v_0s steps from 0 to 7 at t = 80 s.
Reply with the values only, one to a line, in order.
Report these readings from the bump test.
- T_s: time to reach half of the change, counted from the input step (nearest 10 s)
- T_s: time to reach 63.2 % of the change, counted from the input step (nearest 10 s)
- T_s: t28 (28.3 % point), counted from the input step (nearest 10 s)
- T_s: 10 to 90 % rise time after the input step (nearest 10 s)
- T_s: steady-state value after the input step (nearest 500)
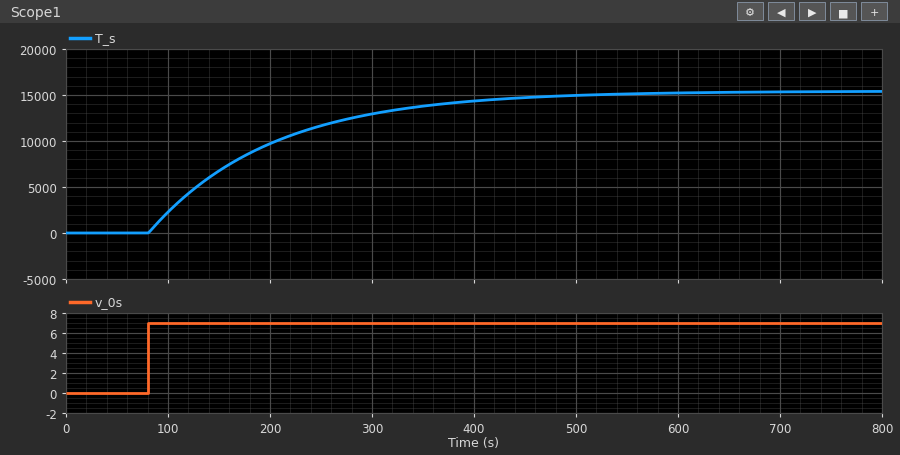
80 s
120 s
40 s
260 s
15500
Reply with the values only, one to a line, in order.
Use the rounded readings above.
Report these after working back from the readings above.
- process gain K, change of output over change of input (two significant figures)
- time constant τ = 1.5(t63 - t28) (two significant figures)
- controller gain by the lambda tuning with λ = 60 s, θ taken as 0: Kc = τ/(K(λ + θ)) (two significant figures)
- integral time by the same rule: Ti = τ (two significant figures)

2200
120 s
0.00091
120 s
